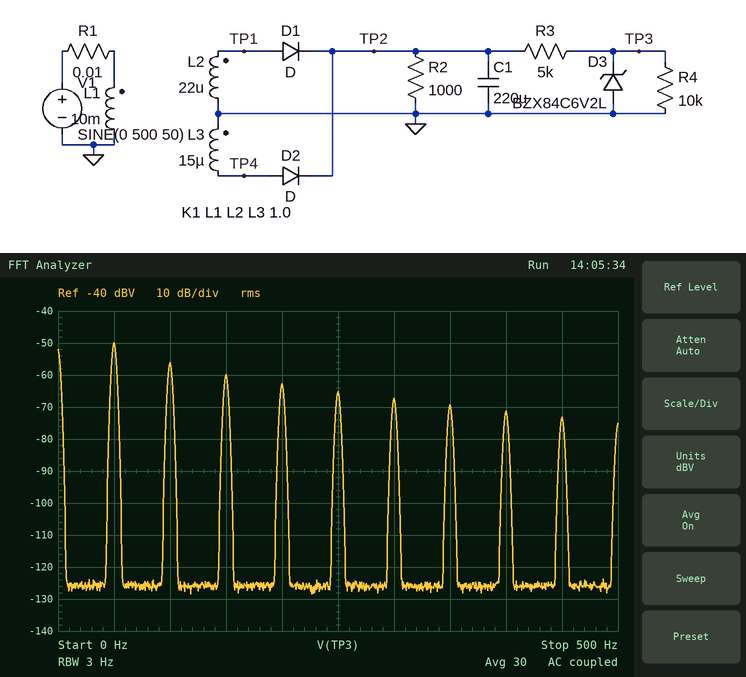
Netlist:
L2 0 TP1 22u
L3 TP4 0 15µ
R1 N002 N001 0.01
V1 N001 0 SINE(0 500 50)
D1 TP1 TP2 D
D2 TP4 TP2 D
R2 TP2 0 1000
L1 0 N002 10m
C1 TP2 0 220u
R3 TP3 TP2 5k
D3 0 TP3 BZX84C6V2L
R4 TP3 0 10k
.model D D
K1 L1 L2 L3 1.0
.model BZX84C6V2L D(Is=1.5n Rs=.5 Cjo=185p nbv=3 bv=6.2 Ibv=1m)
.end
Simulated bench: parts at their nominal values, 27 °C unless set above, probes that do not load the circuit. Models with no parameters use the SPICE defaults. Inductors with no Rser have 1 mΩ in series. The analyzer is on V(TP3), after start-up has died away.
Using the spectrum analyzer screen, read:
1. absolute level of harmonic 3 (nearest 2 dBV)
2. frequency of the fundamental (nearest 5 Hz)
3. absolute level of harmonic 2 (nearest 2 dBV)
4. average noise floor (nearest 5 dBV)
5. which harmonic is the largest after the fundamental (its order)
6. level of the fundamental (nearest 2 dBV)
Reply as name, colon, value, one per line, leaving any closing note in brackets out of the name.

absolute level of harmonic 3: -60 dBV
frequency of the fundamental: 50 Hz
absolute level of harmonic 2: -56 dBV
average noise floor: -125 dBV
which harmonic is the largest after the fundamental: 2
level of the fundamental: -50 dBV
